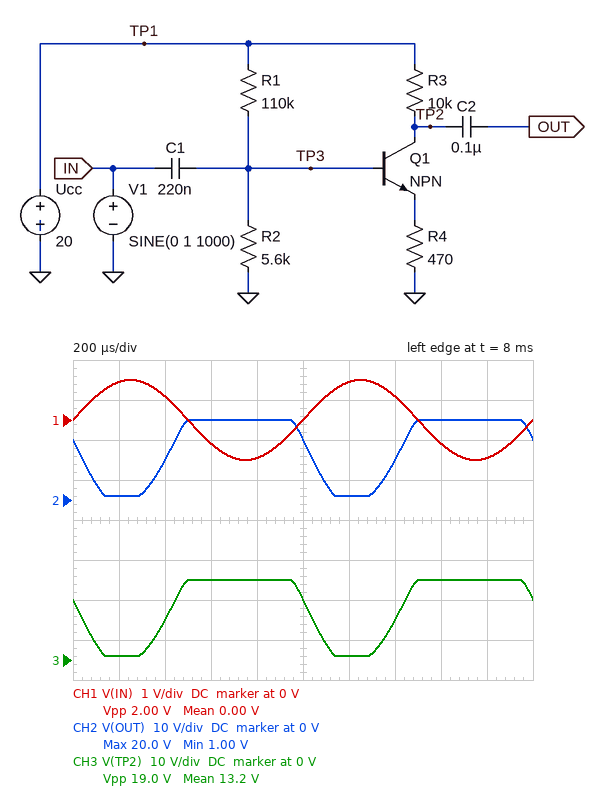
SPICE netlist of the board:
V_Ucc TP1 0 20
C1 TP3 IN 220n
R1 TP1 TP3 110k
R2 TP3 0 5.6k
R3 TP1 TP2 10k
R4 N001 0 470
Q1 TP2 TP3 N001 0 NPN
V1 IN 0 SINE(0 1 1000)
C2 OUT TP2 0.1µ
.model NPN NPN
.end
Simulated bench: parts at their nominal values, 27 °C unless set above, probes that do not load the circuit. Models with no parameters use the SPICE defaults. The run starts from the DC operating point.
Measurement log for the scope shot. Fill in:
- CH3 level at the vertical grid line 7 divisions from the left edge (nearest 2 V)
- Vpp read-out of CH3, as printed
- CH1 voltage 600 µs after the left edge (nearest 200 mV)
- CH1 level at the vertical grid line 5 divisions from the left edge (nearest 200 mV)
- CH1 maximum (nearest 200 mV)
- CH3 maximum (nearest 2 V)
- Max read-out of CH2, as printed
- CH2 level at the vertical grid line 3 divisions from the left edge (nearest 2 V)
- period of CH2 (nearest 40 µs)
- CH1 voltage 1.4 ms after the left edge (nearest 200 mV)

10 V
19.0 V
-600 mV
0 V
1.0 V
20 V
20.0 V
20 V
1.00 ms
600 mV
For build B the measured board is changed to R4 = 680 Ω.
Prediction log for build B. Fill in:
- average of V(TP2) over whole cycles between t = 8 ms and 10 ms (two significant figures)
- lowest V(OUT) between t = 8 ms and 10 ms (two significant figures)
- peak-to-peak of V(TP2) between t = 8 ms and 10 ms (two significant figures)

14 V
3.4 V
17 V
